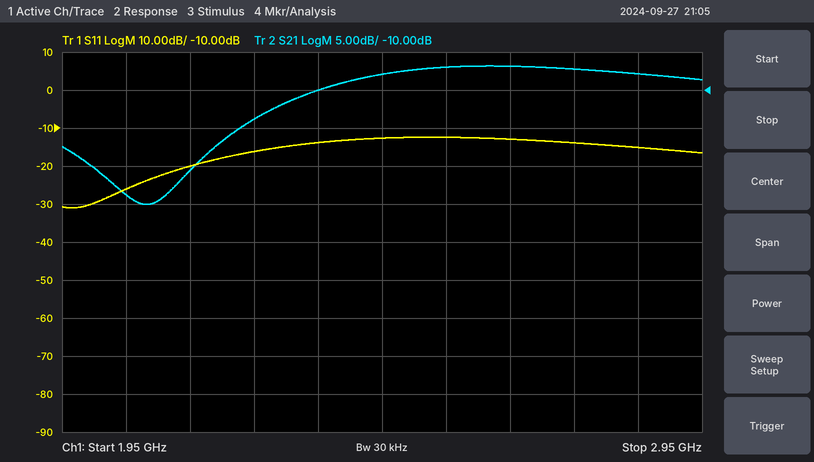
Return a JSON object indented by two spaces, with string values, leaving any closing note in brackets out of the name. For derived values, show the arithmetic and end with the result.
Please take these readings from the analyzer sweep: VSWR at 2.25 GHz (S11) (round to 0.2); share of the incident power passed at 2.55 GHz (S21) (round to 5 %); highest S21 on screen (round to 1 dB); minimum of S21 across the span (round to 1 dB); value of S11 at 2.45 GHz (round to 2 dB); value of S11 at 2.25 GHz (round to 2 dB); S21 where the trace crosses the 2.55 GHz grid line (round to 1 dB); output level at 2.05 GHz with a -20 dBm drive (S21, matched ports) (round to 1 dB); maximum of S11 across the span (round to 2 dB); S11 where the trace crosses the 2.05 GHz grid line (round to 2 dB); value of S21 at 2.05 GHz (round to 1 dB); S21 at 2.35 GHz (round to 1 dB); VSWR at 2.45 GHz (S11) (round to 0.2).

{
  "VSWR at 2.25 GHz (S11)": "|Γ| = 10^(-16/20) = 0.1585; VSWR = (1 + 0.1585)/(1 − 0.1585) ≈ 1.4",
  "share of the incident power passed at 2.55 GHz (S21)": "10^(-7/10) ≈ 20 %",
  "highest S21 on screen": "-7 dB",
  "minimum of S21 across the span": "-25 dB",
  "value of S11 at 2.45 GHz": "-12 dB",
  "value of S11 at 2.25 GHz": "-16 dB",
  "S21 where the trace crosses the 2.55 GHz grid line": "-7 dB",
  "output level at 2.05 GHz with a -20 dBm drive (S21, matched ports)": "-20 dBm + (-24 dB) = -44 dBm",
  "maximum of S11 across the span": "-12 dB",
  "S11 where the trace crosses the 2.05 GHz grid line": "-26 dB",
  "value of S21 at 2.05 GHz": "-24 dB",
  "S21 at 2.35 GHz": "-10 dB",
  "VSWR at 2.45 GHz (S11)": "|Γ| = 10^(-12/20) = 0.2512; VSWR = (1 + 0.2512)/(1 − 0.2512) ≈ 1.67, so 1.6 to the nearest 0.2"
}
